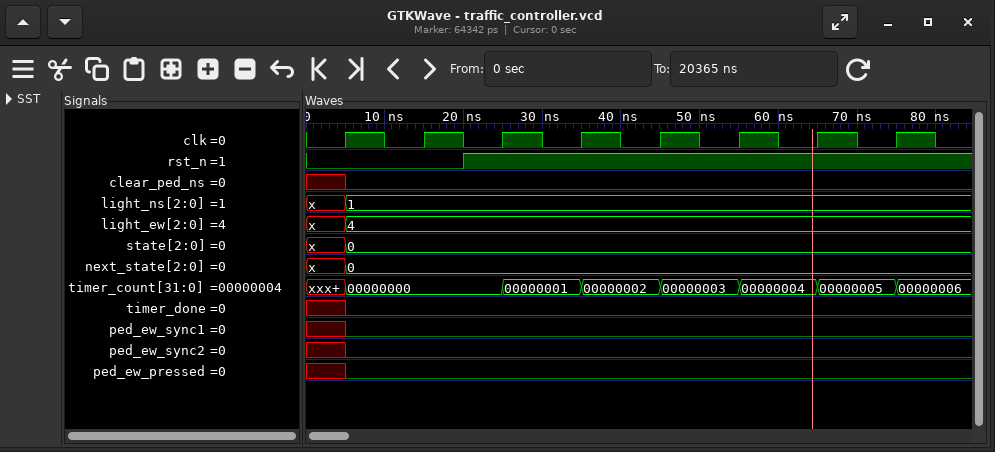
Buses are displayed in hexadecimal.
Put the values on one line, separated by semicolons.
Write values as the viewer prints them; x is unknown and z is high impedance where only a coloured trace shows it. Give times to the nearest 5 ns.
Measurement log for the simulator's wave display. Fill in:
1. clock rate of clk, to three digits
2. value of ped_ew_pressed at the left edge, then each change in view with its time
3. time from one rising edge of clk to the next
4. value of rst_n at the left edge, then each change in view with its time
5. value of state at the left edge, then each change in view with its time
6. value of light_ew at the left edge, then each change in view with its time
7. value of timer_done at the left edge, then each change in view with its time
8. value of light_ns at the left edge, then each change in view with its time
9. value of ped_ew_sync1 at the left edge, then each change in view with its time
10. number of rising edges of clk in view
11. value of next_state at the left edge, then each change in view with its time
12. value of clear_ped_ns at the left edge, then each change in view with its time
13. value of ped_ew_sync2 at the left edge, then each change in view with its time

100 MHz; x, 0 at 5 ns; 10 ns; 0, 1 at 20 ns; x, 0 at 5 ns; x, 4 at 5 ns; x, 0 at 5 ns; x, 1 at 5 ns; x, 0 at 5 ns; 8; x, 0 at 5 ns; x, 0 at 5 ns; x, 0 at 5 ns
